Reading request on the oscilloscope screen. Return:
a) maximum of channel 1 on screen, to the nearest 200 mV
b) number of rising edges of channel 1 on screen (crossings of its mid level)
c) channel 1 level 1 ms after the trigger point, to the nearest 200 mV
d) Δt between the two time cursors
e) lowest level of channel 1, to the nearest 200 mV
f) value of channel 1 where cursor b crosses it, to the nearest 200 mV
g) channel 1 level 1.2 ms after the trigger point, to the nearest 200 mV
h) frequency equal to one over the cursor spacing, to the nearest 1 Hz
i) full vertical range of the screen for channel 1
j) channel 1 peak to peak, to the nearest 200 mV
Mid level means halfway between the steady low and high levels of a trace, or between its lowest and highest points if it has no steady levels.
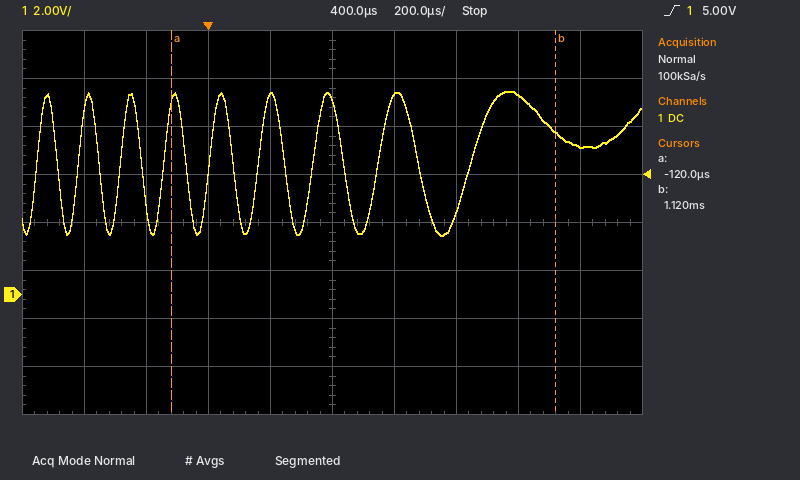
8.4 V
9
8.4 V
1.24 ms
2.4 V
6.8 V
6.2 V
806 Hz
16 V
6.0 V
